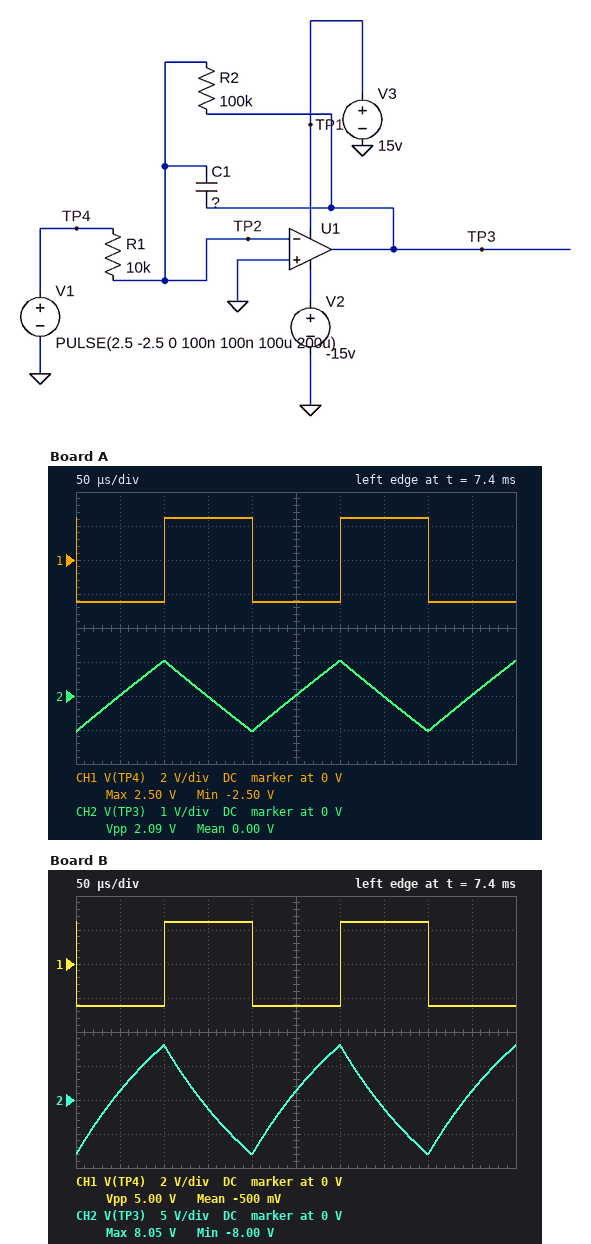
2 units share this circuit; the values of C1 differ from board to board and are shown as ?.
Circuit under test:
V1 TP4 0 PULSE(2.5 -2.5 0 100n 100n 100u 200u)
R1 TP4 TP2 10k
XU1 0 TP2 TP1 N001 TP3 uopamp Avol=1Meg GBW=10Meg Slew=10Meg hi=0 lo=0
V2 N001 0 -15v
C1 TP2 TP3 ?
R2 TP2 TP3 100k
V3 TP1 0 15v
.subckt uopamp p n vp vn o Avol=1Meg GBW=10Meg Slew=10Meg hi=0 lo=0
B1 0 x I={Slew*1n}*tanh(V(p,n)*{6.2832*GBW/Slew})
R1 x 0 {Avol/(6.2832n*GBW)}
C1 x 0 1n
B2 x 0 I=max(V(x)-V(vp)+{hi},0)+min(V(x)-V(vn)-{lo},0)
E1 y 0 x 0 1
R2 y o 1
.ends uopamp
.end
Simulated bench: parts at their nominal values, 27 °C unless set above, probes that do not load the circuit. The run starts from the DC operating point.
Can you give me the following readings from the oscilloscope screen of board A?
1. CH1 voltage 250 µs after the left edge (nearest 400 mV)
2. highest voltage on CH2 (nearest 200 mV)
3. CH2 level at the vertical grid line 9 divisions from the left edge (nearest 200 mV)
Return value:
-2.4 V
1.0 V
0 V
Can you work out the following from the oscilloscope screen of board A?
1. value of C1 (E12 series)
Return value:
12 nF
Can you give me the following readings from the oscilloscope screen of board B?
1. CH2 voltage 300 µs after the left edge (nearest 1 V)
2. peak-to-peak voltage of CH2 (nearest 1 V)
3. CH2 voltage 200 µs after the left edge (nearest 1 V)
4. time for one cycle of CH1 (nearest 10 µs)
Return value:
8 V
16 V
-8 V
200 µs
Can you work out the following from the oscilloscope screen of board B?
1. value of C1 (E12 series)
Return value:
1.5 nF
